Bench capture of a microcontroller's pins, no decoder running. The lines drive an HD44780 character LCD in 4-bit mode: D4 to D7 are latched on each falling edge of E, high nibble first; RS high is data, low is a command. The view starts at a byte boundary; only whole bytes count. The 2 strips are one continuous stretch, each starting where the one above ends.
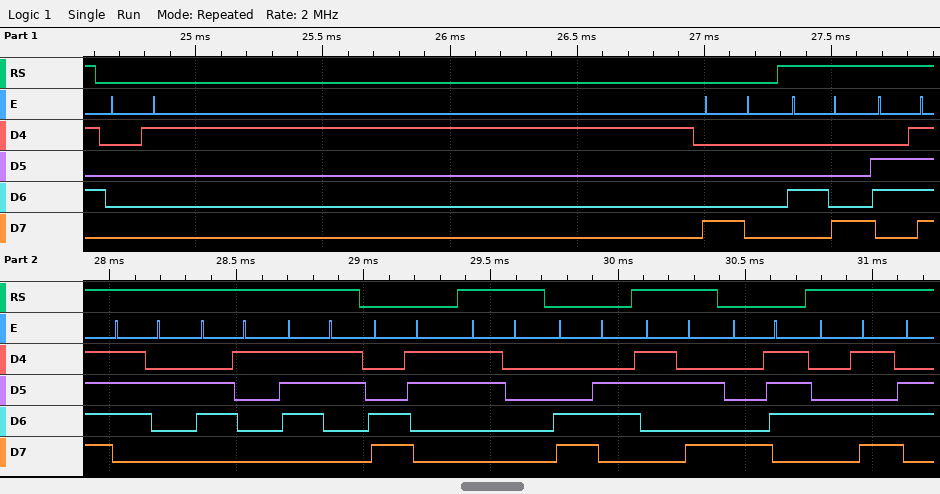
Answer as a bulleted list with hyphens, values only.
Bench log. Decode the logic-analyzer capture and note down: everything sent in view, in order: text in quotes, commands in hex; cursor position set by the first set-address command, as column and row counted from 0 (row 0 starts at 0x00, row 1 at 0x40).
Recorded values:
- 0x01 0x80 "Horas" 0xC3 "0" 0xC6 ":" 0x87 "M"
- column 0, row 0
